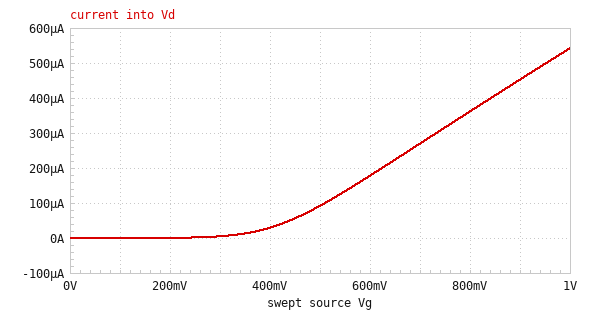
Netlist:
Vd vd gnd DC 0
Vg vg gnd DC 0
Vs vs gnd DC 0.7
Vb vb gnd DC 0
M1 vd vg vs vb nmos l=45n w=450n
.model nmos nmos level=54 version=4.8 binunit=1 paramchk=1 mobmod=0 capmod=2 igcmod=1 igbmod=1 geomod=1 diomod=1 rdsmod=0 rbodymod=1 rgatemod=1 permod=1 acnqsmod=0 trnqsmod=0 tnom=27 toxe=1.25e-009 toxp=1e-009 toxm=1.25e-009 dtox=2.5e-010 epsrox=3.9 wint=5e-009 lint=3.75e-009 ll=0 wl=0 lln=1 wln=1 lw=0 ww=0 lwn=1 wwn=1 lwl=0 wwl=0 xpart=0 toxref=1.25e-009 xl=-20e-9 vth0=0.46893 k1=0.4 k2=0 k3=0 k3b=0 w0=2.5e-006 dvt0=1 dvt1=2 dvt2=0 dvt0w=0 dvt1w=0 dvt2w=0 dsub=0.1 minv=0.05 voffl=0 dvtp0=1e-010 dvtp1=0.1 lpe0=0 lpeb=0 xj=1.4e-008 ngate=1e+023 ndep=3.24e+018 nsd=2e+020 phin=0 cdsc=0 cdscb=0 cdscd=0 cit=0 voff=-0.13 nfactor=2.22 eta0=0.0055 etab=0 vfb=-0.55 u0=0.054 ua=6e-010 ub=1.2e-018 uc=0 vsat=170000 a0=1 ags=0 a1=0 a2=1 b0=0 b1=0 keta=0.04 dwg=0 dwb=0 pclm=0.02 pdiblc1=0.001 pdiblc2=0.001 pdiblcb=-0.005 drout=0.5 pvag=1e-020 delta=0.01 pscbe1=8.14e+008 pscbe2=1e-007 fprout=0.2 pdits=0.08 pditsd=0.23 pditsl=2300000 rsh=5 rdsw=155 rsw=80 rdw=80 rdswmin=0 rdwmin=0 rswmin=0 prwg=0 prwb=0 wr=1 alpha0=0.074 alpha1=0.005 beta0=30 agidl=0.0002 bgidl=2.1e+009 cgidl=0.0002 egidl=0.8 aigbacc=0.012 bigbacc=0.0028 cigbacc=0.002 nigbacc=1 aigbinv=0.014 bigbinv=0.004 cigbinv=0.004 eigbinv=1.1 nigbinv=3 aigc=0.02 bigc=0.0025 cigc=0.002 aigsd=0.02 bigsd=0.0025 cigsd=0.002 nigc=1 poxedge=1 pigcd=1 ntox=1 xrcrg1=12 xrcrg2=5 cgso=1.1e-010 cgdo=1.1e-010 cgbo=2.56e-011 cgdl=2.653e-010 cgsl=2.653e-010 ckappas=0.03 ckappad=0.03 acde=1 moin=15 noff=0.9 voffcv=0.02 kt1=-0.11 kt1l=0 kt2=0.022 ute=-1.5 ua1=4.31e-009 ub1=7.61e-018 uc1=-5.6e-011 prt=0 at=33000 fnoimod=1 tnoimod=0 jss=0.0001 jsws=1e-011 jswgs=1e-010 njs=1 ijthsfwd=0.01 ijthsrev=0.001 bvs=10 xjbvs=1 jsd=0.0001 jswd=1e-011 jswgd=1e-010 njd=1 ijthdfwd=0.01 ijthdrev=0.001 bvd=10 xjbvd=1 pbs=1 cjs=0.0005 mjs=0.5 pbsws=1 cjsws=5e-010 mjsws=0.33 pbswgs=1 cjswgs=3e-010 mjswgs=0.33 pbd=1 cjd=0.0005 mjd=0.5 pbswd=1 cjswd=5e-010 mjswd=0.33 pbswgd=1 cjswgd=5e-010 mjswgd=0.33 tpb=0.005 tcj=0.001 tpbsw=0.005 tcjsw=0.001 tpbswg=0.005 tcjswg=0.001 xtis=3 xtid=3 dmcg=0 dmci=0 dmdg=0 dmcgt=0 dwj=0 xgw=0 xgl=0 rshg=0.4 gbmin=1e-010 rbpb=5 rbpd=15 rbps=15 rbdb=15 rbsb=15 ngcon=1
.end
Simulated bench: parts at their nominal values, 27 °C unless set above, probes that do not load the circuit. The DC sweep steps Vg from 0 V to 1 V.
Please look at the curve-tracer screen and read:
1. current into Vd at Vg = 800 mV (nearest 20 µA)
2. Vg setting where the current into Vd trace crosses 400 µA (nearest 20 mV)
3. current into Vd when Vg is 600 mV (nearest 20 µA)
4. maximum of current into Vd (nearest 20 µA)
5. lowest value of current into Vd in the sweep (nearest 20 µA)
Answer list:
360 µA
840 mV
180 µA
540 µA
0 A
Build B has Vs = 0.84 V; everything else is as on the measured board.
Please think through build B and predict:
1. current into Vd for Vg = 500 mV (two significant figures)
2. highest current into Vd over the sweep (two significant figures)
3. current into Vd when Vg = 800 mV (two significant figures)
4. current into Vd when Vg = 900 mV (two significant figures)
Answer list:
110 µA
570 µA
380 µA
480 µA
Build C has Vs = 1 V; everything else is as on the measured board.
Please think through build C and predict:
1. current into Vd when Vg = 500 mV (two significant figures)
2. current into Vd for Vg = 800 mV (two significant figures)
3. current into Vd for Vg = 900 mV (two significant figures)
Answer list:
130 µA
410 µA
500 µA
